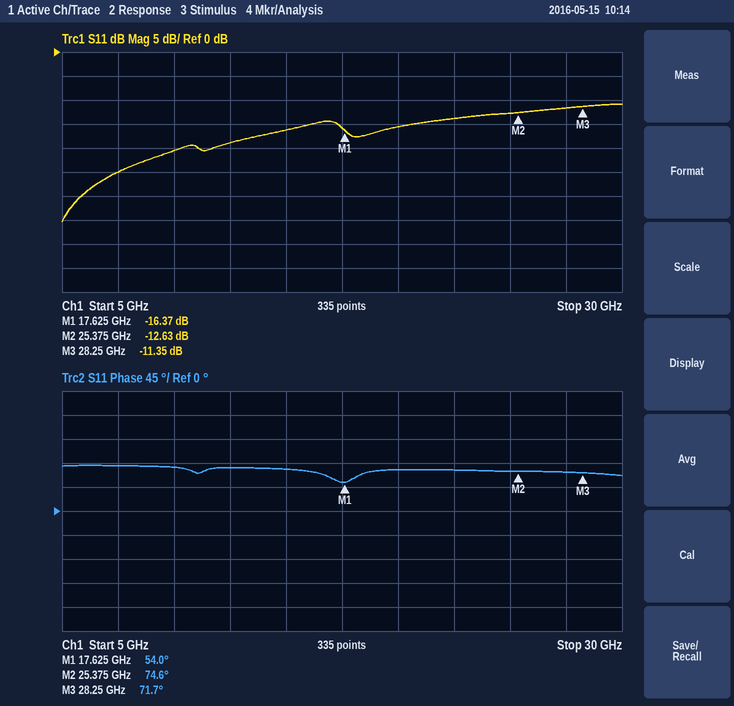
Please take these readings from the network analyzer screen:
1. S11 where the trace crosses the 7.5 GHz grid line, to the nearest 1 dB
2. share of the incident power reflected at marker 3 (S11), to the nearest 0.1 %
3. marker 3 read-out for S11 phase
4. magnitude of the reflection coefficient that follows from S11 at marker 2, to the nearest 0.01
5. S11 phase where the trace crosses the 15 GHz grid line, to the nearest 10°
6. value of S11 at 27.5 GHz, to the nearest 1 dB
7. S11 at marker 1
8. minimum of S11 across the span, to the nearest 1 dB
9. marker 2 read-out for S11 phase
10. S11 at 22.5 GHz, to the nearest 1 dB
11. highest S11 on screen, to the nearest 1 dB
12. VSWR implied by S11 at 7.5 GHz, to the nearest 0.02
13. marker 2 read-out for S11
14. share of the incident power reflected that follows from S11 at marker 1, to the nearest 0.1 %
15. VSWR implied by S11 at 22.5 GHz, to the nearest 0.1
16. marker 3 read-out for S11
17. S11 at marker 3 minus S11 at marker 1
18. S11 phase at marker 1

-25 dB
7.3 %
71.7°
0.23
80°
-12 dB
-16.37 dB
-35 dB
74.6°
-14 dB
-11 dB
1.12
-12.63 dB
2.3 %
1.5
-11.35 dB
5.02 dB
54.0°
